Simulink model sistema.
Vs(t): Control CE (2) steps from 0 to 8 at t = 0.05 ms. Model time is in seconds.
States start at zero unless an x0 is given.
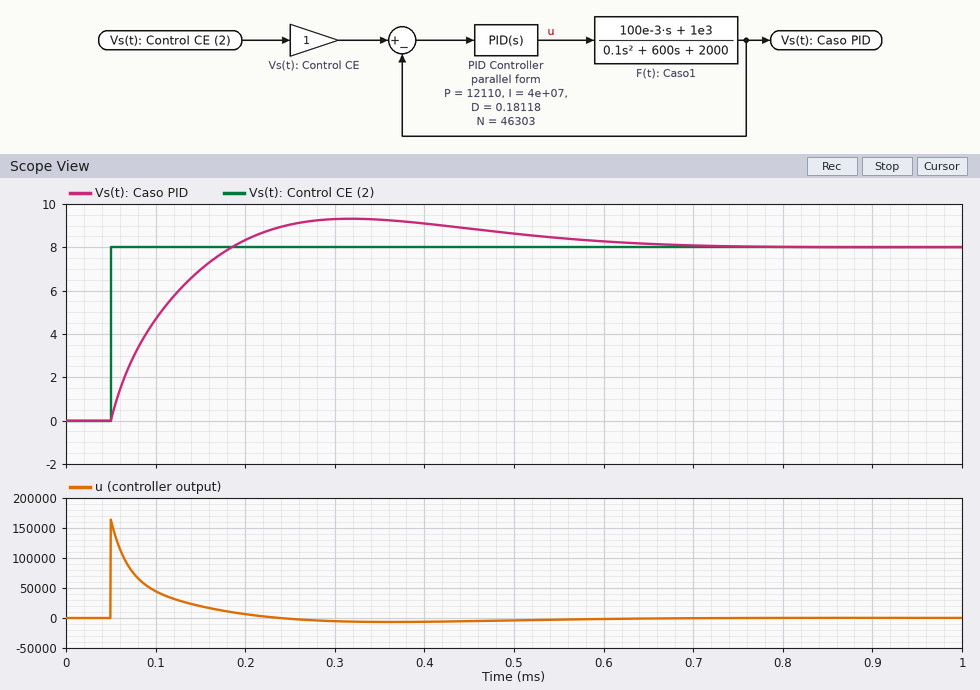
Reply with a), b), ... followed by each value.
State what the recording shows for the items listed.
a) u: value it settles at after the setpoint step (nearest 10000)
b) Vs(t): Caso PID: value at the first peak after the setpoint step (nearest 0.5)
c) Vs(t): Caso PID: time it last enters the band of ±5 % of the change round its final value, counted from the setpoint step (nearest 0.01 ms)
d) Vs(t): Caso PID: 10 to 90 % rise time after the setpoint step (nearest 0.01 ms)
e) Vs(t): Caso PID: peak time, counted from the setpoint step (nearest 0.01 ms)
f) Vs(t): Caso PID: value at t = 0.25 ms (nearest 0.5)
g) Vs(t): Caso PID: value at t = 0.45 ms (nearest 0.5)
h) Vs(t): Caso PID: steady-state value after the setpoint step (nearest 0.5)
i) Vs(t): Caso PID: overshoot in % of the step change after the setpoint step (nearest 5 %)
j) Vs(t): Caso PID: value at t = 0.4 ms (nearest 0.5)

a) 0
b) 9.5
c) 0.51 ms
d) 0.10 ms
e) 0.27 ms
f) 9.0
g) 9.0
h) 8.0
i) 15 %
j) 9.0
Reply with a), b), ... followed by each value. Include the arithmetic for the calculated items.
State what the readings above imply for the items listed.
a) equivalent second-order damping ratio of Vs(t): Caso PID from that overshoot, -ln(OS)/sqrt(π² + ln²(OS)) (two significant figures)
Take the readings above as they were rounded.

a) ln(0.15) = -1.897; 1.897 / sqrt(9.870 + 3.599) = 0.52
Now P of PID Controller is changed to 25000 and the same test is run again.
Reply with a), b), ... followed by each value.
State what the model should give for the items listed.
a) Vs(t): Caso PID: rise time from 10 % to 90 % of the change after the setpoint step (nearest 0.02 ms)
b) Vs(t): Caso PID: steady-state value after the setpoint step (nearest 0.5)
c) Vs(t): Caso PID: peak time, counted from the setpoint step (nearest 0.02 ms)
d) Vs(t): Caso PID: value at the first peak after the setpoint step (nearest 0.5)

a) 0.06 ms
b) 8.0
c) 0.18 ms
d) 8.5
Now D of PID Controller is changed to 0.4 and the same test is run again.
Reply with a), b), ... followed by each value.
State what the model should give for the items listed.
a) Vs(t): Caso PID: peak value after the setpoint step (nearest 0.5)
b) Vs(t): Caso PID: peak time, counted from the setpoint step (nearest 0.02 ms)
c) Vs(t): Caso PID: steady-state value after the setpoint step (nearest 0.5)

a) 9.0
b) 0.30 ms
c) 8.0
